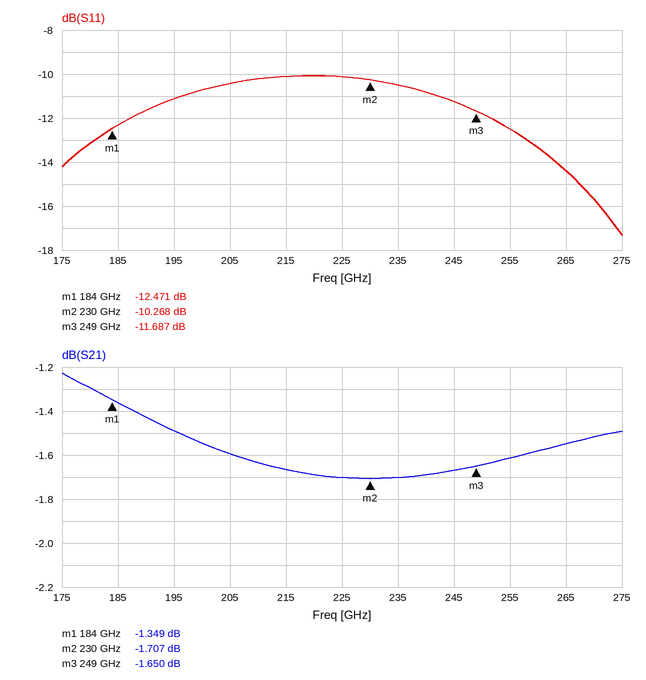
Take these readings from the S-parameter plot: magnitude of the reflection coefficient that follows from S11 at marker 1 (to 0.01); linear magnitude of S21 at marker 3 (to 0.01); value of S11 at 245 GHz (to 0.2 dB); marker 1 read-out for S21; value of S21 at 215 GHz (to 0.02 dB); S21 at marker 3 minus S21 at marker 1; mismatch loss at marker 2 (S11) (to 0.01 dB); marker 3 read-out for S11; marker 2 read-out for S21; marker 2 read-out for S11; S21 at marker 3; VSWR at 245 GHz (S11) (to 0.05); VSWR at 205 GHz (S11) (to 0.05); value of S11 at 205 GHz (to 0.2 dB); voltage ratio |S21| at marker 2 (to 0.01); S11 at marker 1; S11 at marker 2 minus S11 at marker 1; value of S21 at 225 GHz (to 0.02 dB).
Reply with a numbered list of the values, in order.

1. 0.24
2. 0.83
3. -11.2 dB
4. -1.349 dB
5. -1.66 dB
6. -0.301 dB
7. 0.43 dB
8. -11.687 dB
9. -1.707 dB
10. -10.268 dB
11. -1.650 dB
12. 1.75
13. 1.85
14. -10.4 dB
15. 0.82
16. -12.471 dB
17. 2.203 dB
18. -1.70 dB
